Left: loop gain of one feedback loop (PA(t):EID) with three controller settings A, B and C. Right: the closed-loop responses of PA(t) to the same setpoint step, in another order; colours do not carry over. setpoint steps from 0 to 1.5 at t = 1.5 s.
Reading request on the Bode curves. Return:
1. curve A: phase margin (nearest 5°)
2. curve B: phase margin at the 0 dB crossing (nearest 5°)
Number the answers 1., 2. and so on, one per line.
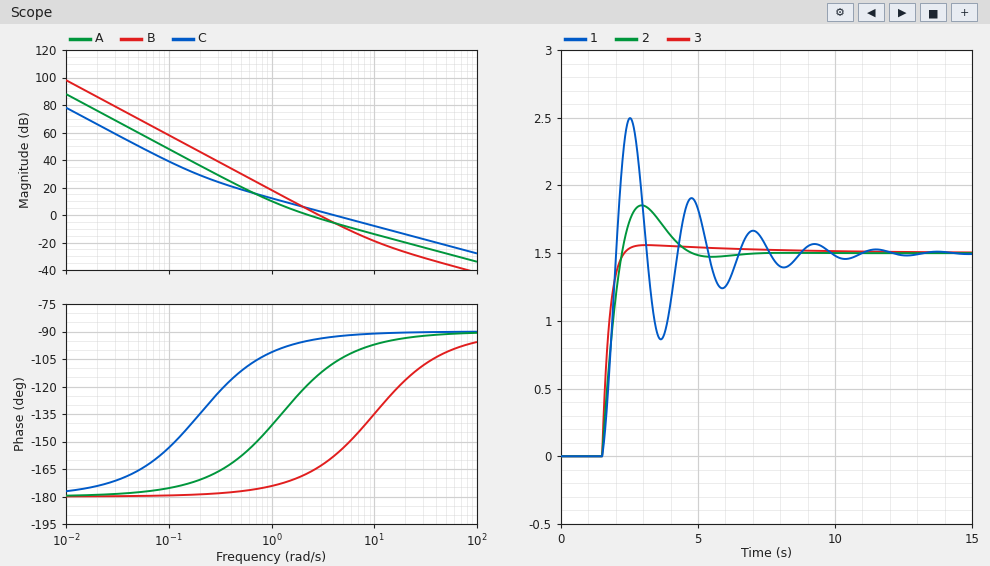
1. 60°
2. 15°
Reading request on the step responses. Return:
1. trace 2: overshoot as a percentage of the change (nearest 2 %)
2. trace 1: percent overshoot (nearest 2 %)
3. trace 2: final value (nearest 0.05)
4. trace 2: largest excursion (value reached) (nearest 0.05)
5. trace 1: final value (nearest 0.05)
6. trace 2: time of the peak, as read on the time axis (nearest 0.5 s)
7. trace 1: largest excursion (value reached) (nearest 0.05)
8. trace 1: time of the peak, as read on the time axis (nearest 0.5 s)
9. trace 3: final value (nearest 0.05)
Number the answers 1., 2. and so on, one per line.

1. 24 %
2. 66 %
3. 1.50
4. 1.85
5. 1.50
6. 3.0 s
7. 2.50
8. 2.5 s
9. 1.50
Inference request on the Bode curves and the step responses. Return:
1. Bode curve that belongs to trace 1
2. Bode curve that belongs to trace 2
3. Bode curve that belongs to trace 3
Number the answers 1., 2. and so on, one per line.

1. B
2. A
3. C
